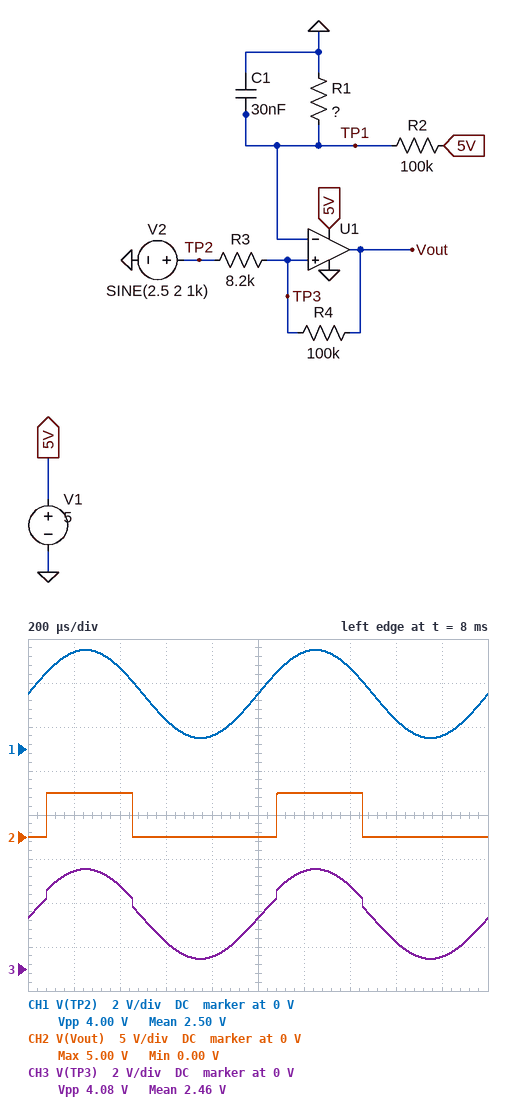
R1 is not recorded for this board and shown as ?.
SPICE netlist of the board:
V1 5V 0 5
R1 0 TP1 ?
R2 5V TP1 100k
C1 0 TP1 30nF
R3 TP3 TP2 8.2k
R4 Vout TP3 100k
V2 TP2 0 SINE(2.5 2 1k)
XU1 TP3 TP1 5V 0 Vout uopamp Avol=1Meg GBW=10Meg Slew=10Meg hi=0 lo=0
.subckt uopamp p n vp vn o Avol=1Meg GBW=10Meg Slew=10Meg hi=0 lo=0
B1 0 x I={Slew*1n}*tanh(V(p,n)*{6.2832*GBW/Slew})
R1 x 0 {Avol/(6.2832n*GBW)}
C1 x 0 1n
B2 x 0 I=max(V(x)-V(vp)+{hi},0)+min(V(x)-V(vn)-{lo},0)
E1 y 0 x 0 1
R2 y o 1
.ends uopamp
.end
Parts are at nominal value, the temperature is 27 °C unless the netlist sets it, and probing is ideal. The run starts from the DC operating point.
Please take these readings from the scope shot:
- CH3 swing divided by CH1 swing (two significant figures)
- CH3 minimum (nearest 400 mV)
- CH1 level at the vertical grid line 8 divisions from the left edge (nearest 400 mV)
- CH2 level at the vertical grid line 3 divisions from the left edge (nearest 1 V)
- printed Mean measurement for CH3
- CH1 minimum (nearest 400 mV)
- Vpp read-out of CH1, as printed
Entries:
1.0
400 mV
1.2 V
0 V
2.46 V
400 mV
4.00 V
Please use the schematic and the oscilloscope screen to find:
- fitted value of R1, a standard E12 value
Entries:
180 kΩ
